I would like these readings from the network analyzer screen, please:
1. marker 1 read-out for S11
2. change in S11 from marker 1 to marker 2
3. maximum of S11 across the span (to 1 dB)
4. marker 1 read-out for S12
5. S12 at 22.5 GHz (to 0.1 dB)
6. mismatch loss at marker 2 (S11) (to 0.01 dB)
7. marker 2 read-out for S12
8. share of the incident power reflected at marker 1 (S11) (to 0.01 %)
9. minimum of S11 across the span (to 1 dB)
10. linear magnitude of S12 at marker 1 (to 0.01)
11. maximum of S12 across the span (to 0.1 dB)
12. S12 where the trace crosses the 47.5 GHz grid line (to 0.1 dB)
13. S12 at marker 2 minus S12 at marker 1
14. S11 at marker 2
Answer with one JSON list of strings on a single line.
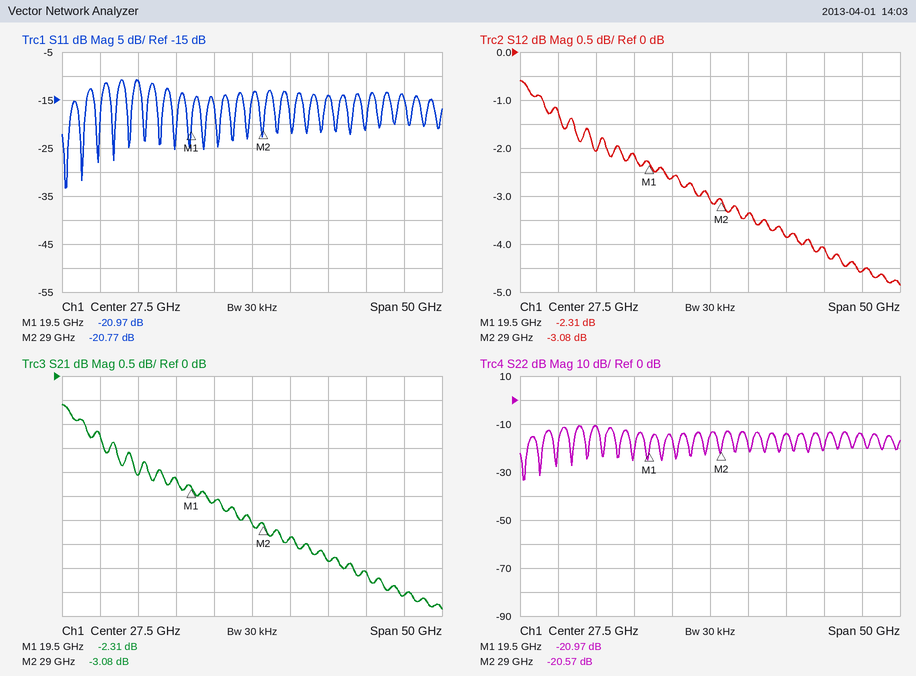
["-20.97 dB", "0.20 dB", "-11 dB", "-2.31 dB", "-2.6 dB", "0.04 dB", "-3.08 dB", "0.80 %", "-33 dB", "0.77", "-0.6 dB", "-4.6 dB", "-0.77 dB", "-20.77 dB"]
